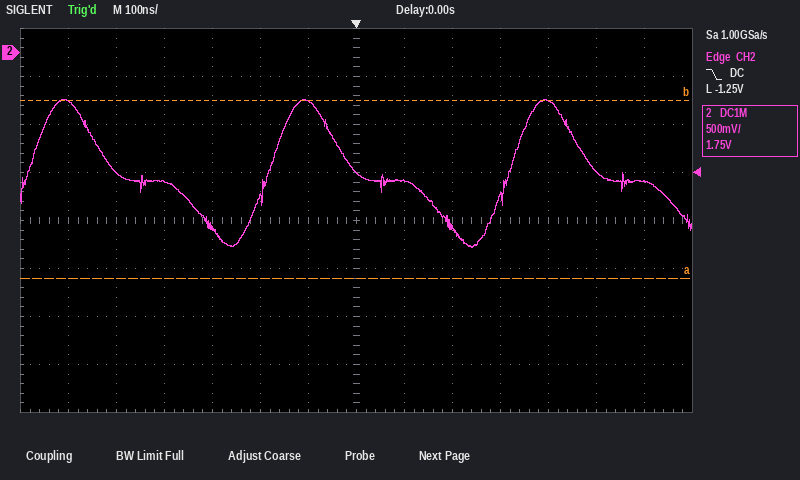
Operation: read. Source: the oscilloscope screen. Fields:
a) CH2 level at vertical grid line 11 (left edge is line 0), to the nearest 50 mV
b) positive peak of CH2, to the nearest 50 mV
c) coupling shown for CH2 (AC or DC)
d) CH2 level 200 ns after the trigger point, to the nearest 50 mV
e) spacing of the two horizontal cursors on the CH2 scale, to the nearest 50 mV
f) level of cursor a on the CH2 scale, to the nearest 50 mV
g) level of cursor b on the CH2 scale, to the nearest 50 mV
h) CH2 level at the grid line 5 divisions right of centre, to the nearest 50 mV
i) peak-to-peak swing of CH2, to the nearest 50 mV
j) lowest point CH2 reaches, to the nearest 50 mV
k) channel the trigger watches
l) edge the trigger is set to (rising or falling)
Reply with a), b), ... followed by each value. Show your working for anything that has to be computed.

a) -500 mV
b) -500 mV
c) DC
d) -1.80 V
e) 1.85 V
f) -2.35 V
g) -500 mV
h) -1.25 V
i) -500 mV − (-2.05 V) = 1.55 V
j) -2.05 V
k) CH2
l) falling
